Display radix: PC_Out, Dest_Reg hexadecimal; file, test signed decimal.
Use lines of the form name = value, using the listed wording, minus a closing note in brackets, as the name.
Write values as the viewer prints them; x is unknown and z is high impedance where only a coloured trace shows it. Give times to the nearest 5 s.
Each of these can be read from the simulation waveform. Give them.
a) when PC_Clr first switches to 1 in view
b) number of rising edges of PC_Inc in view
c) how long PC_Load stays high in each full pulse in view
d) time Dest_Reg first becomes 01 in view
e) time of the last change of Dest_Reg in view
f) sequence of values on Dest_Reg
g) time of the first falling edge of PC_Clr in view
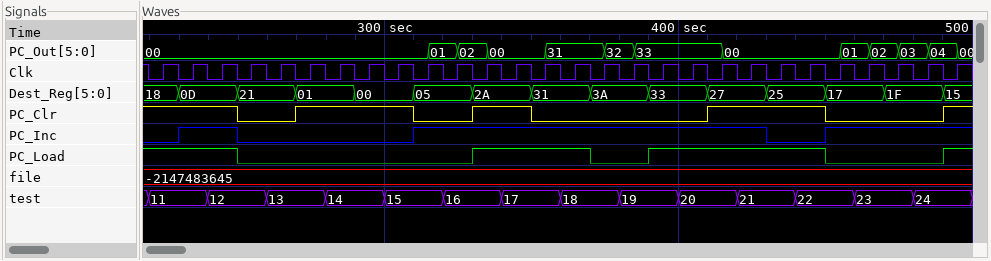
when PC_Clr first switches to 1 in view = 270 s
number of rising edges of PC_Inc in view = 3
how long PC_Load stays high in each full pulse in view = 40 s, 60 s
time Dest_Reg first becomes 01 in view = 270 s
time of the last change of Dest_Reg in view = 490 s
sequence of values on Dest_Reg = 18, 0D, 21, 01, 00, 05, 2A, 31, 3A, 33, 27, 25, 17, 1F, 15
time of the first falling edge of PC_Clr in view = 250 s
